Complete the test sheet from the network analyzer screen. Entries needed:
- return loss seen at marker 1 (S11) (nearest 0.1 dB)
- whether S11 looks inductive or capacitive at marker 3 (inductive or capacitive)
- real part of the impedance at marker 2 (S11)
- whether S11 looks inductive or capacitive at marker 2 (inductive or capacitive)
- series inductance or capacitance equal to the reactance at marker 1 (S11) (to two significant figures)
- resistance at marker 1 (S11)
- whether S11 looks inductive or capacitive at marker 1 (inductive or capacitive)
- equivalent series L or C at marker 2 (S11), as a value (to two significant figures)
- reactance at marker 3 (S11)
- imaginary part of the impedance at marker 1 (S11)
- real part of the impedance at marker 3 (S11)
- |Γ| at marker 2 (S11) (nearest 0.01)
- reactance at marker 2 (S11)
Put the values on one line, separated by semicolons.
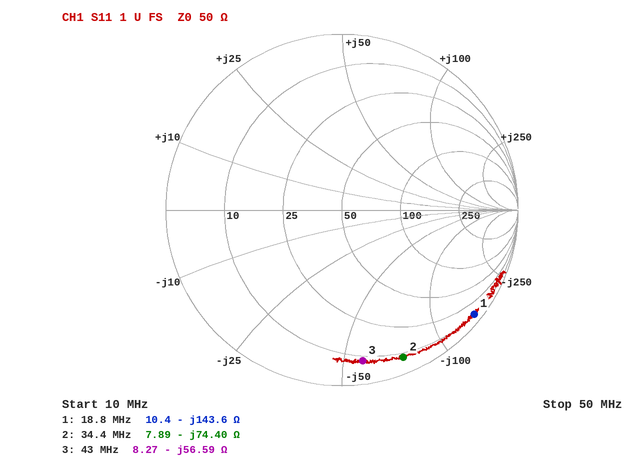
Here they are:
0.4 dB; capacitive; 7.89 Ω; capacitive; 59 pF; 10.4 Ω; capacitive; 62 pF; -56.59 Ω; -143.6 Ω; 8.27 Ω; 0.91; -74.40 Ω
